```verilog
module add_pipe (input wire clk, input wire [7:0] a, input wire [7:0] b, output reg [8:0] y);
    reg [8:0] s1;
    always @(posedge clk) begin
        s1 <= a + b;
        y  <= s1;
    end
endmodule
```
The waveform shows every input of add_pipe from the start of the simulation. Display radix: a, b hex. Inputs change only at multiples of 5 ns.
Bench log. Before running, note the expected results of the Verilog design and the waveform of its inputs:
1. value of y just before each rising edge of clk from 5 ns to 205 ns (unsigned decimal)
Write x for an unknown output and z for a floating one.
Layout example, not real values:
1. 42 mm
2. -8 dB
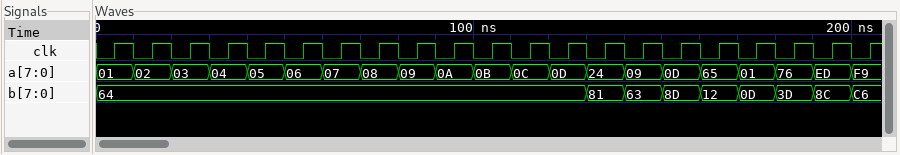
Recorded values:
1. x, x, 101, 102, 103, 104, 105, 106, 107, 108, 109, 110, 111, 112, 113, 165, 108, 154, 119, 14, 179
